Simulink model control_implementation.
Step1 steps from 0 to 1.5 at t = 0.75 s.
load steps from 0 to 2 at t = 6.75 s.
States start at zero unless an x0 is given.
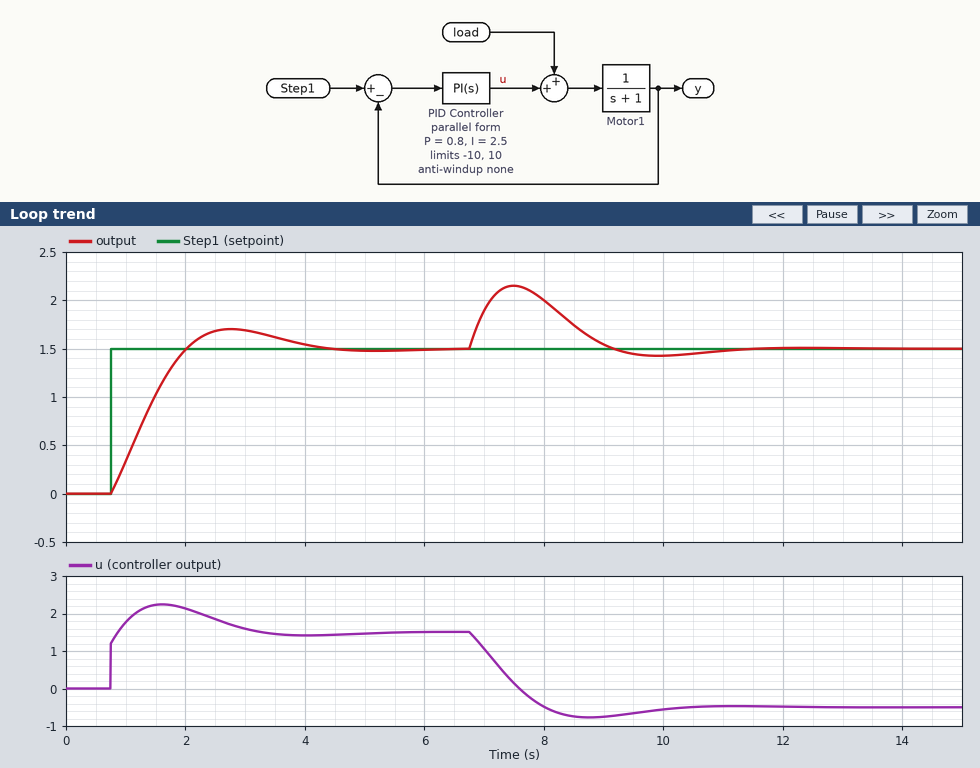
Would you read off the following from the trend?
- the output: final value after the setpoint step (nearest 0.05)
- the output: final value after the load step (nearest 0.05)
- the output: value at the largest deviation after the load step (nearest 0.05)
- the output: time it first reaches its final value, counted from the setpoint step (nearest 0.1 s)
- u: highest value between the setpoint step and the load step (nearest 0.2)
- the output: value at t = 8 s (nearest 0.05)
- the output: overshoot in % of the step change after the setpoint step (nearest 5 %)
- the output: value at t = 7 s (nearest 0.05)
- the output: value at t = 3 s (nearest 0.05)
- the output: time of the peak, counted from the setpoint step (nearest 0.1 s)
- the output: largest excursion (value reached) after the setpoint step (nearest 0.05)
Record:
1.50
1.50
2.15
1.3 s
2.2
2.00
15 %
1.90
1.70
2.0 s
1.70
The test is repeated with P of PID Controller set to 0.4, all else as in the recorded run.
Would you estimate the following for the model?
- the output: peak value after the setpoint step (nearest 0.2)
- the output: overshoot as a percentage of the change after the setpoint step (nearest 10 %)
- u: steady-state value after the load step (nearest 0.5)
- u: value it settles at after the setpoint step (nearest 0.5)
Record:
1.8
20 %
-0.5
1.5
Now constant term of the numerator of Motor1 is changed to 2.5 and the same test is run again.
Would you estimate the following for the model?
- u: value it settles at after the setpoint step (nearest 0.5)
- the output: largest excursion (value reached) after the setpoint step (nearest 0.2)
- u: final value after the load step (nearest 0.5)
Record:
0.5
1.8
-1.5
